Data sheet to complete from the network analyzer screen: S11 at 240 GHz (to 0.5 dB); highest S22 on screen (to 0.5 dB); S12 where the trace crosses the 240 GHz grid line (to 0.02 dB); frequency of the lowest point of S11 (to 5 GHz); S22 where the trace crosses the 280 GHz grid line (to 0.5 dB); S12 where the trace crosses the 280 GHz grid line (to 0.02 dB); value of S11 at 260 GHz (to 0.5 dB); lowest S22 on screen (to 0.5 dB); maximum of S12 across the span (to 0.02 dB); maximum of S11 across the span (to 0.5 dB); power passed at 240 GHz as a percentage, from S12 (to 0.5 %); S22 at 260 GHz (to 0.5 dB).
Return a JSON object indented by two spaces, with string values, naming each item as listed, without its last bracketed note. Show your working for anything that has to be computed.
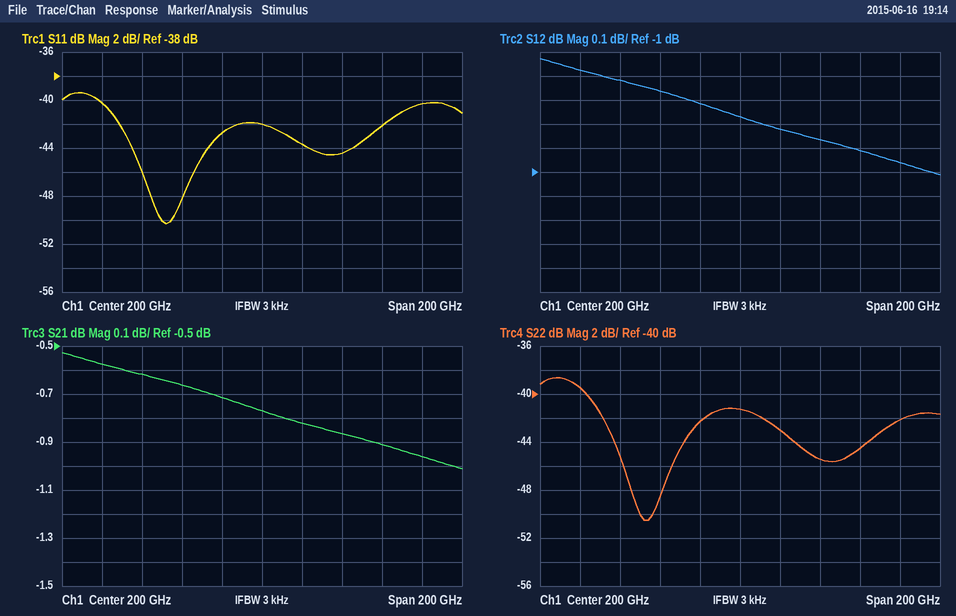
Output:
{
  "S11 at 240 GHz": "-44.5 dB",
  "highest S22 on screen": "-38.5 dB",
  "S12 where the trace crosses the 240 GHz grid line": "-0.86 dB",
  "frequency of the lowest point of S11": "150 GHz",
  "S22 where the trace crosses the 280 GHz grid line": "-42.0 dB",
  "S12 where the trace crosses the 280 GHz grid line": "-0.96 dB",
  "value of S11 at 260 GHz": "-42.0 dB",
  "lowest S22 on screen": "-50.5 dB",
  "maximum of S12 across the span": "-0.52 dB",
  "maximum of S11 across the span": "-39.5 dB",
  "power passed at 240 GHz as a percentage, from S12": "10^(-0.86/10) ≈ 82.0 %",
  "S22 at 260 GHz": "-44.5 dB"
}
